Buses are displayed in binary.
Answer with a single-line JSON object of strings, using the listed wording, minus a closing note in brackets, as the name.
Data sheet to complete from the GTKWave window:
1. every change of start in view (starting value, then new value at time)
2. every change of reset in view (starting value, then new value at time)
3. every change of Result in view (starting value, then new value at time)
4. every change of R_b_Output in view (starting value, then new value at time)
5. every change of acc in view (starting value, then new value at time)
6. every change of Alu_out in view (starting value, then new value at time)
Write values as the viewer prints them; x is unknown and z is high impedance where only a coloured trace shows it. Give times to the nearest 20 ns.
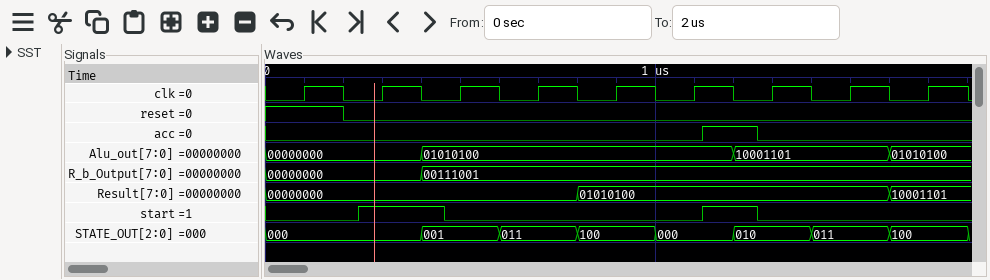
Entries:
{"every change of start in view": "0, 1 at 240 ns, 0 at 460 ns, 1 at 1120 ns, 0 at 1260 ns", "every change of reset in view": "1, 0 at 200 ns", "every change of Result in view": "00000000, 01010100 at 800 ns, 10001101 at 1600 ns", "every change of R_b_Output in view": "00000000, 00111001 at 400 ns", "every change of acc in view": "0, 1 at 1120 ns, 0 at 1260 ns", "every change of Alu_out in view": "00000000, 01010100 at 400 ns, 10001101 at 1200 ns, 01010100 at 1600 ns"}
